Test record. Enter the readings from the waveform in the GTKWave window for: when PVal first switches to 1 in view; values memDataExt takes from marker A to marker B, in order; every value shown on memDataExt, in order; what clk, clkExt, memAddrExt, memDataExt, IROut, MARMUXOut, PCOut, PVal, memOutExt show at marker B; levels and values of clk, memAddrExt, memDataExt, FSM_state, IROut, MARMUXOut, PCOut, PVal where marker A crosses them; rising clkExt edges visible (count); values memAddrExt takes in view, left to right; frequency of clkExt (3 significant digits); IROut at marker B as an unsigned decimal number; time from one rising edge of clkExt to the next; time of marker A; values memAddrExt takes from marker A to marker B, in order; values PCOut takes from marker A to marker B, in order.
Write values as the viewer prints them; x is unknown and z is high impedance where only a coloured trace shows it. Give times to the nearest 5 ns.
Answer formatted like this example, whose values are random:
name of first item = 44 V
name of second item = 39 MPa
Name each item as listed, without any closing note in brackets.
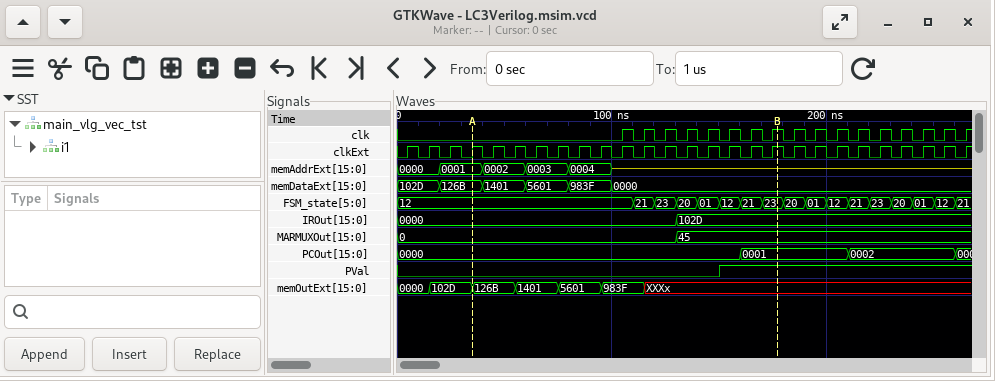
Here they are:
when PVal first switches to 1 in view = 150 ns
values memDataExt takes from marker A to marker B, in order = 126B, 1401, 5601, 983F, 0000
every value shown on memDataExt, in order = 102D, 126B, 1401, 5601, 983F, 0000
what clk, clkExt, memAddrExt, memDataExt, IROut, MARMUXOut, PCOut, PVal, memOutExt show at marker B = clk=1, clkExt=1, memAddrExt=z, memDataExt=0000, IROut=102D, MARMUXOut=45, PCOut=0001, PVal=1, memOutExt=XXXx
levels and values of clk, memAddrExt, memDataExt, FSM_state, IROut, MARMUXOut, PCOut, PVal where marker A crosses them = clk=0, memAddrExt=0001, memDataExt=126B, FSM_state=12, IROut=0000, MARMUXOut=0, PCOut=0000, PVal=0
rising clkExt edges visible = 27
values memAddrExt takes in view, left to right = 0000, 0001, 0002, 0003, 0004, z
frequency of clkExt = 100 MHz
IROut at marker B as an unsigned decimal number = 4141
time from one rising edge of clkExt to the next = 10 ns
time of marker A = 35 ns
values memAddrExt takes from marker A to marker B, in order = 0001, 0002, 0003, 0004, z
values PCOut takes from marker A to marker B, in order = 0000, 0001
